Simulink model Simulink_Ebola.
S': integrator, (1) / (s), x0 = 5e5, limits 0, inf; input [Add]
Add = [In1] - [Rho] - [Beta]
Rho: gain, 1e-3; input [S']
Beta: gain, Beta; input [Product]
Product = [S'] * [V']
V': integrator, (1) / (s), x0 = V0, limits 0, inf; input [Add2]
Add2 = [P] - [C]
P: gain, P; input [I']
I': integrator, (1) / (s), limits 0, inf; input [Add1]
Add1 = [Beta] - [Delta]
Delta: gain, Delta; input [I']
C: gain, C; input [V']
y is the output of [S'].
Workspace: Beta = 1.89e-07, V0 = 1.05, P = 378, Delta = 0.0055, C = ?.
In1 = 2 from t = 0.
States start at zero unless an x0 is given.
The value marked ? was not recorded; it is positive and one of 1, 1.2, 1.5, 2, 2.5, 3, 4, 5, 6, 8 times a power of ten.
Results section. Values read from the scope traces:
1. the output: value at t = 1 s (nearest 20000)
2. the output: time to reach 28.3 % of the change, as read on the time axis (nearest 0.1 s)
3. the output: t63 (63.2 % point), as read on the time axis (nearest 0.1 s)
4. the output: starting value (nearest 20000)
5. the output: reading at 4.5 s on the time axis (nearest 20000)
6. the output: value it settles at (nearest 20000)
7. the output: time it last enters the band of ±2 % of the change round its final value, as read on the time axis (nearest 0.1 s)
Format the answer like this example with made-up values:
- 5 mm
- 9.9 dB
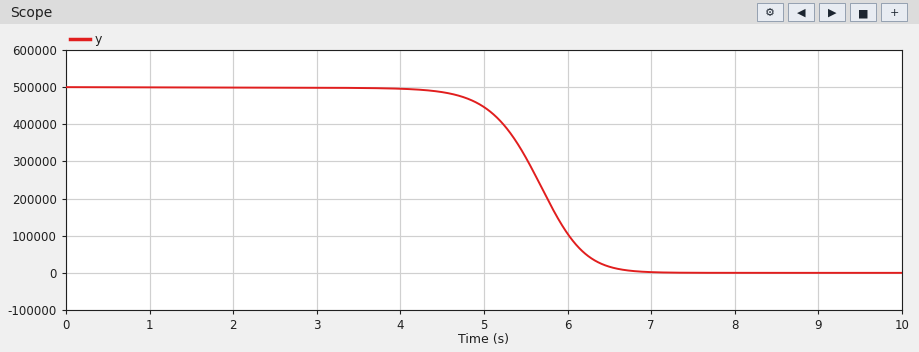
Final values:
- 500000
- 5.4 s
- 5.8 s
- 500000
- 480000
- 0
- 6.6 s
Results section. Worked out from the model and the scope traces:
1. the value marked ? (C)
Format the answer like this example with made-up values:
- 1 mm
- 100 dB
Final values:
- 8
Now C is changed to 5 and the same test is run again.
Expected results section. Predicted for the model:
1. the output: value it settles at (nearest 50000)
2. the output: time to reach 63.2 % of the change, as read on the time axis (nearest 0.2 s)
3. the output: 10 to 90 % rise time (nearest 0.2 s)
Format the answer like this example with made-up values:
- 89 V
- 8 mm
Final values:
- 0
- 4.6 s
- 1.0 s
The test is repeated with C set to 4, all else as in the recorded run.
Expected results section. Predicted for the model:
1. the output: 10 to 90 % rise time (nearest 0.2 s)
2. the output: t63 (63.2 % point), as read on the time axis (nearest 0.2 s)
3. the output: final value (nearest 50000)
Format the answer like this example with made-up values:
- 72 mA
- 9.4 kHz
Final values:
- 0.8 s
- 4.2 s
- 0
